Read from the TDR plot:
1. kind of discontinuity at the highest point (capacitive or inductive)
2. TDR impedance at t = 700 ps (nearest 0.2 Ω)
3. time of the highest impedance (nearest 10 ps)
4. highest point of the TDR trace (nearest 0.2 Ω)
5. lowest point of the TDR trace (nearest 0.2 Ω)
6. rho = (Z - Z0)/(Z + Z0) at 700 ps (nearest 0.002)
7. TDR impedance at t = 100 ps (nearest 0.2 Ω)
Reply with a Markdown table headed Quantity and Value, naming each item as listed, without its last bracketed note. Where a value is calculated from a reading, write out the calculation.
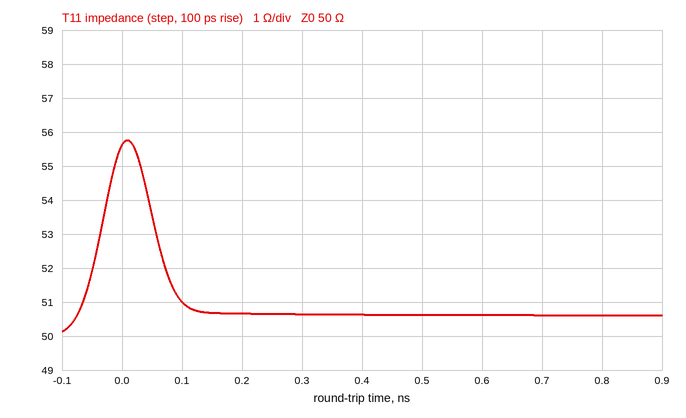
| Quantity | Value |
|---|---|
| kind of discontinuity at the highest point | inductive |
| TDR impedance at t = 700 ps | 50.6 Ω |
| time of the highest impedance | 10 ps |
| highest point of the TDR trace | 55.8 Ω |
| lowest point of the TDR trace | 50.2 Ω |
| rho = (Z - Z0)/(Z + Z0) at 700 ps | (50.6 − 50)/(50.6 + 50) ≈ +0.006 |
| TDR impedance at t = 100 ps | 51.0 Ω |
